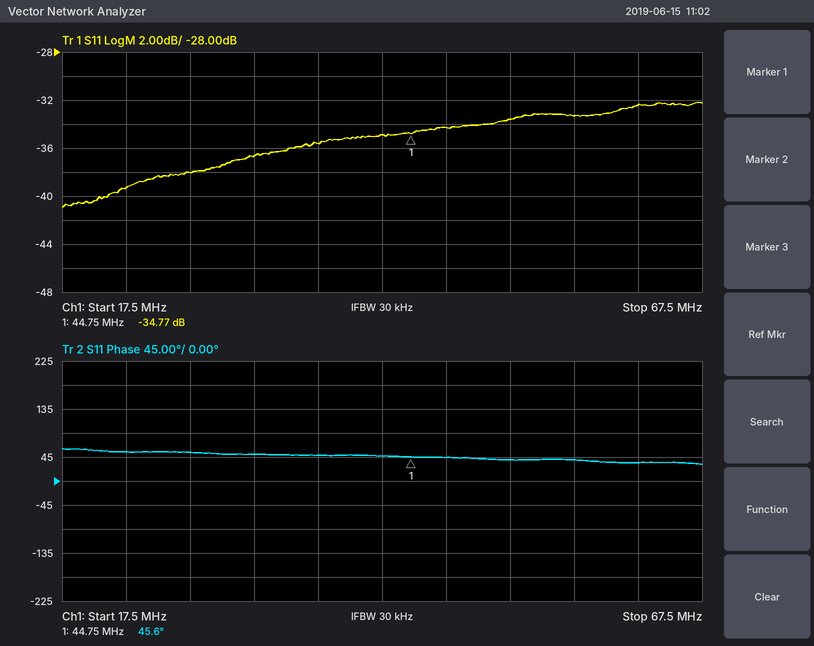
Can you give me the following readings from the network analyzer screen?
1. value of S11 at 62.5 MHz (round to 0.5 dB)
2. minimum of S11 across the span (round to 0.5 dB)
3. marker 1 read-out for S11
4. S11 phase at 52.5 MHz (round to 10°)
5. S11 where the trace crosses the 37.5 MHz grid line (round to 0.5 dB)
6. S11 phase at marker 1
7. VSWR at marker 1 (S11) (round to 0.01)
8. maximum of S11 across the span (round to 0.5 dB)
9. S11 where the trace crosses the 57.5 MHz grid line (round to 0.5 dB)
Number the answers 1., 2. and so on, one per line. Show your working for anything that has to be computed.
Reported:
1. -32.5 dB
2. -41.0 dB
3. -34.77 dB
4. 40°
5. -35.5 dB
6. 45.6°
7. (1 + 0.0183)/(1 − 0.0183) ≈ 1.04
8. -32.0 dB
9. -33.5 dB
